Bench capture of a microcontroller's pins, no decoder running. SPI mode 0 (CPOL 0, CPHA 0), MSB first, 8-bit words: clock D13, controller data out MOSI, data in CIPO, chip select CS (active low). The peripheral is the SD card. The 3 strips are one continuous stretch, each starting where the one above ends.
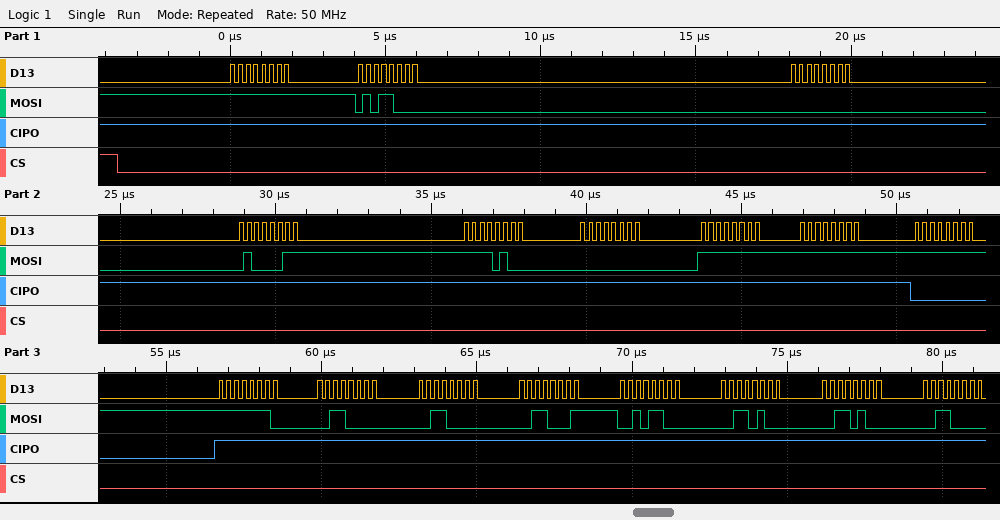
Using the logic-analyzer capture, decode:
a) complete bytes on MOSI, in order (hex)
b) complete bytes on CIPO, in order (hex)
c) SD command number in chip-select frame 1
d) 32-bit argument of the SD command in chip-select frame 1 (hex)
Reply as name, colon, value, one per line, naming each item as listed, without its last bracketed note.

complete bytes on MOSI, in order: FF 58 00 43 F4 00 FF FF FF FE 30 30 31 2C 34 34 30
complete bytes on CIPO, in order: FF FF FF FF FF FF FF FF 00 FF FF FF FF FF FF FF FF
SD command number in chip-select frame 1: CMD24
32-bit argument of the SD command in chip-select frame 1: 0x0043F400
